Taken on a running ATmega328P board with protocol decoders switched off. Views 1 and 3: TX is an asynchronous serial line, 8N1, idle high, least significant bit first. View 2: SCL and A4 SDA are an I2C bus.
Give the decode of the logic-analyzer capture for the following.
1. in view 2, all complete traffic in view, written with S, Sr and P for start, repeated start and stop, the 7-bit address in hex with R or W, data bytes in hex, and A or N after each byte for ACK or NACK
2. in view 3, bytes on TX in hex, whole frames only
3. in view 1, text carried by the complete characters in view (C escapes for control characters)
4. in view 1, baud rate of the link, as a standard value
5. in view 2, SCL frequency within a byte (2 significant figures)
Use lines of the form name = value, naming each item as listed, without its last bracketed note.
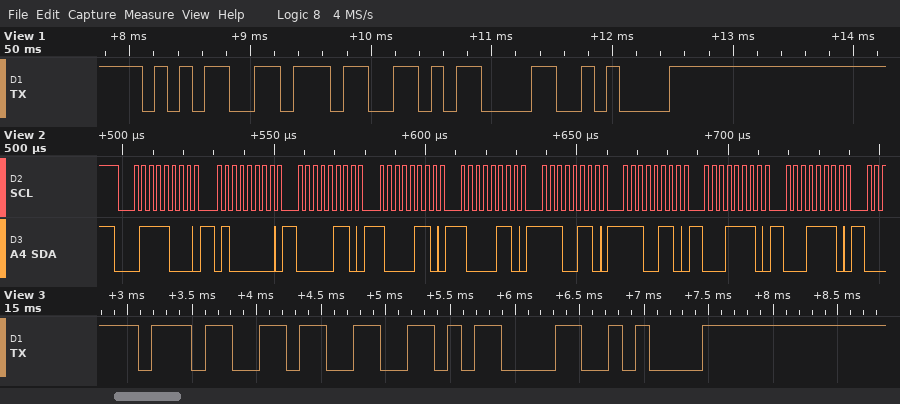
in view 2, all complete traffic in view, written with S, Sr and P for start, repeated start and stop, the 7-bit address in hex with R or W, data bytes in hex, and A or N after each byte for ACK or NACK = S 3CW A 40 A 06 A 86 A 86 A E6 A E6 A 1E A 1E A
in view 3, bytes on TX in hex, whole frames only = 37 33 0D 0A
in view 1, text carried by the complete characters in view = "57\r\n"
in view 1, baud rate of the link, as a standard value = 9600 baud
in view 2, SCL frequency within a byte = 400 kHz
